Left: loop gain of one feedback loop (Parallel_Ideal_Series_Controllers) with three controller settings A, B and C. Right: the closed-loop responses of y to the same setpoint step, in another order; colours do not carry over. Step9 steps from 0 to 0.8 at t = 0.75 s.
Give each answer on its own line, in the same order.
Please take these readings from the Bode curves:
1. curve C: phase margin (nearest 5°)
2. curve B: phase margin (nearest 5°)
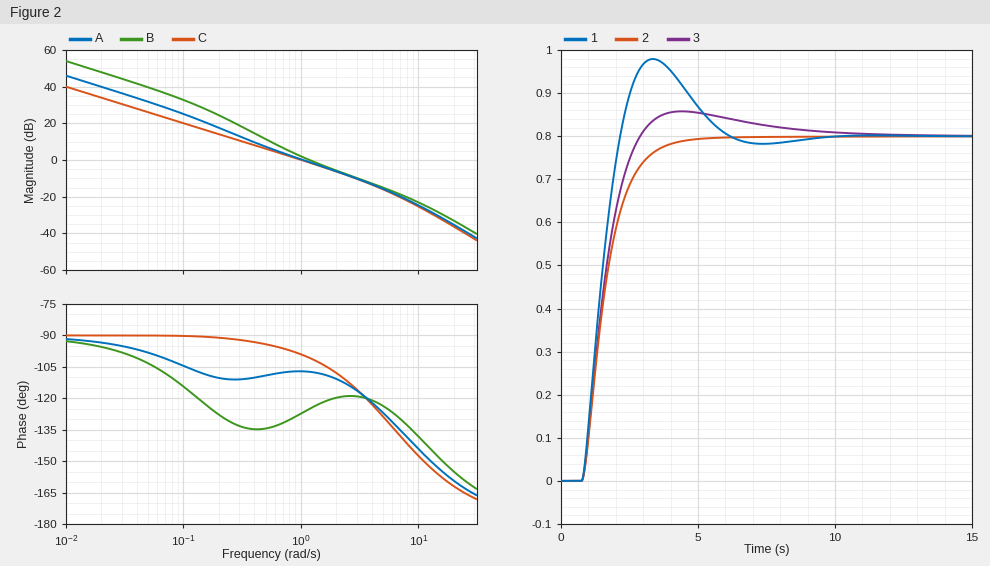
80°
55°
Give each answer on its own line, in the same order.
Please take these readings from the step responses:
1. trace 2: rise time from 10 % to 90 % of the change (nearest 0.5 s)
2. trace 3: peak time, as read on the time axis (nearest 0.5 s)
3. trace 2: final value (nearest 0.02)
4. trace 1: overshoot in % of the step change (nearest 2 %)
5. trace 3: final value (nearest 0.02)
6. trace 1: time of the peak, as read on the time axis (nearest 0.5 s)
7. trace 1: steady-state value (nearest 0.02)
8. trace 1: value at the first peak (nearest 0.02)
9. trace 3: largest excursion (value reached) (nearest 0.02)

2.0 s
4.5 s
0.80
22 %
0.80
3.5 s
0.80
0.98
0.86
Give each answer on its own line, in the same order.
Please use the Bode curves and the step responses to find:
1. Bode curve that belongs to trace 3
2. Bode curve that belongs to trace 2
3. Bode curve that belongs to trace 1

A
C
B
